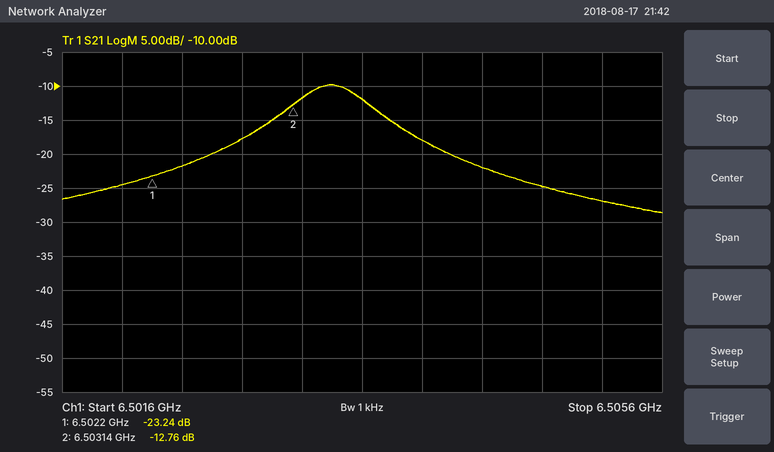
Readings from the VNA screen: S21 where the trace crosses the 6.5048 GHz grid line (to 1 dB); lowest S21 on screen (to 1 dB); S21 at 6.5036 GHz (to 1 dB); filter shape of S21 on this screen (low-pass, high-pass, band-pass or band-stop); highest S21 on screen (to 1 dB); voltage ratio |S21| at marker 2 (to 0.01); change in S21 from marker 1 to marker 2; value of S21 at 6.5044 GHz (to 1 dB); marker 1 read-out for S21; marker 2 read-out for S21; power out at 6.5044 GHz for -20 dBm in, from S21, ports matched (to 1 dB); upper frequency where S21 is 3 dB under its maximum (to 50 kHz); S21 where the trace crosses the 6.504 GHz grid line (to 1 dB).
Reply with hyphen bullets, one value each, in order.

- -25 dB
- -29 dB
- -12 dB
- band-pass
- -10 dB
- 0.23
- 10.48 dB
- -22 dB
- -23.24 dB
- -12.76 dB
- -42 dBm
- 6.50365 GHz
- -18 dB
